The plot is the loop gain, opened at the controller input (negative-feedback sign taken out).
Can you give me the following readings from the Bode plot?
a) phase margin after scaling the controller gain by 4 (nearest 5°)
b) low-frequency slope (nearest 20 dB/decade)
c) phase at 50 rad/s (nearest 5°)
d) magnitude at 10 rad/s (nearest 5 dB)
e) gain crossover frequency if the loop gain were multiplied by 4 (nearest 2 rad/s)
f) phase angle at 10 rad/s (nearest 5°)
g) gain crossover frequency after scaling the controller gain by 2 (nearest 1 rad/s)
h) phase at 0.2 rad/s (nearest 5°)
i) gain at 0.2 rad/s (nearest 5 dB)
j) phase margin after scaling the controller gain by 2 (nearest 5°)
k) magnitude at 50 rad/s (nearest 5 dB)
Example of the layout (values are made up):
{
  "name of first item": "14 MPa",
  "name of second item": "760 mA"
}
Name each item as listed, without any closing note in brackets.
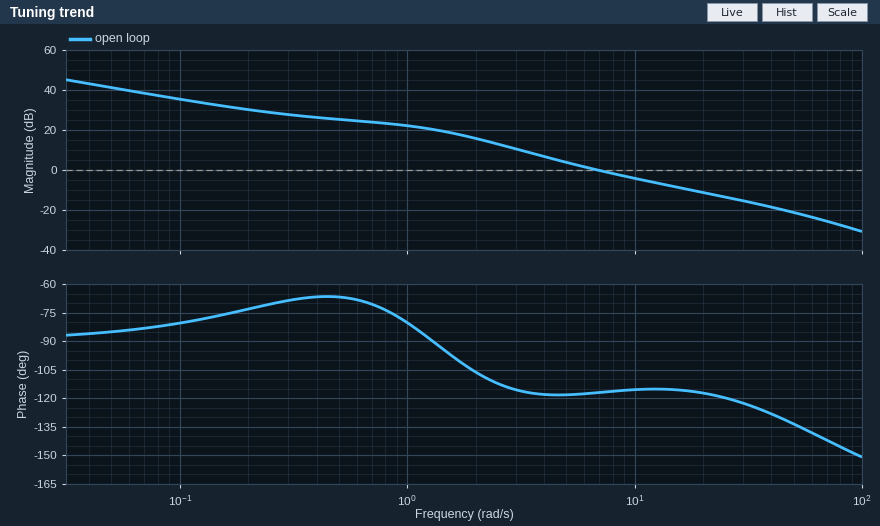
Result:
{
  "phase margin after scaling the controller gain by 4": "60°",
  "low-frequency slope": "-20 dB/decade",
  "phase at 50 rad/s": "-135°",
  "magnitude at 10 rad/s": "-5 dB",
  "gain crossover frequency if the loop gain were multiplied by 4": "22 rad/s",
  "phase angle at 10 rad/s": "-115°",
  "gain crossover frequency after scaling the controller gain by 2": "12 rad/s",
  "phase at 0.2 rad/s": "-75°",
  "gain at 0.2 rad/s": "30 dB",
  "phase margin after scaling the controller gain by 2": "65°",
  "magnitude at 50 rad/s": "-20 dB"
}
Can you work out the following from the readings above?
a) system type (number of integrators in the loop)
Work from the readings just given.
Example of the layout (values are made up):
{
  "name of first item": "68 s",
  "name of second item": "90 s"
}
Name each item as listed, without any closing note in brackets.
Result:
{
  "system type": "1"
}
